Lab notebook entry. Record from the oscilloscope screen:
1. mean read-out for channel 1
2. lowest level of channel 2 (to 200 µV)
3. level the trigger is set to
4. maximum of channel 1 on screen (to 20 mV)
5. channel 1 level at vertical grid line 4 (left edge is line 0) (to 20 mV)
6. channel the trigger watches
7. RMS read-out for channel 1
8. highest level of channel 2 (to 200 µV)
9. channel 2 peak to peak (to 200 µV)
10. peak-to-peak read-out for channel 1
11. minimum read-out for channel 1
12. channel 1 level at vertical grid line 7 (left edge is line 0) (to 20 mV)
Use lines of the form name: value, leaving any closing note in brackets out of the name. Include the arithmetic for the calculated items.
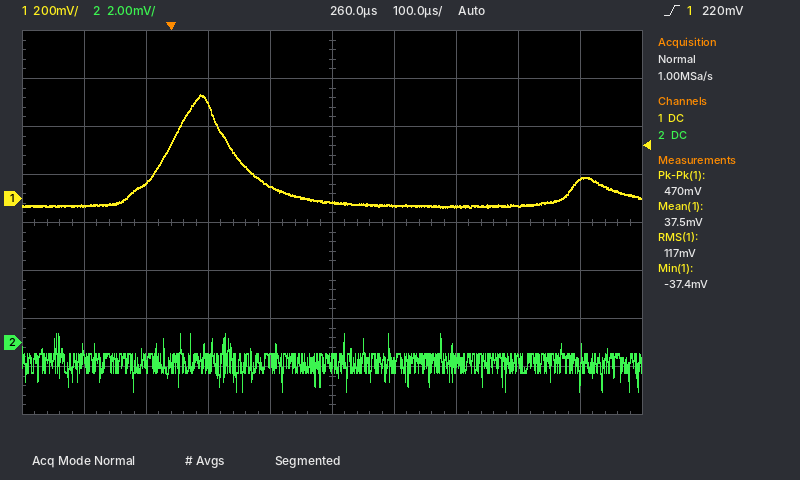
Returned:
mean read-out for channel 1: 37.5 mV
lowest level of channel 2: -2.0 mV
level the trigger is set to: 220 mV
maximum of channel 1 on screen: 440 mV
channel 1 level at vertical grid line 4 (left edge is line 0): 60 mV
channel the trigger watches: channel 1
RMS read-out for channel 1: 117 mV
highest level of channel 2: 400 µV
channel 2 peak to peak: 400 µV − (-2.0 mV) = 2.4 mV
peak-to-peak read-out for channel 1: 470 mV
minimum read-out for channel 1: -37.4 mV
channel 1 level at vertical grid line 7 (left edge is line 0): -40 mV
